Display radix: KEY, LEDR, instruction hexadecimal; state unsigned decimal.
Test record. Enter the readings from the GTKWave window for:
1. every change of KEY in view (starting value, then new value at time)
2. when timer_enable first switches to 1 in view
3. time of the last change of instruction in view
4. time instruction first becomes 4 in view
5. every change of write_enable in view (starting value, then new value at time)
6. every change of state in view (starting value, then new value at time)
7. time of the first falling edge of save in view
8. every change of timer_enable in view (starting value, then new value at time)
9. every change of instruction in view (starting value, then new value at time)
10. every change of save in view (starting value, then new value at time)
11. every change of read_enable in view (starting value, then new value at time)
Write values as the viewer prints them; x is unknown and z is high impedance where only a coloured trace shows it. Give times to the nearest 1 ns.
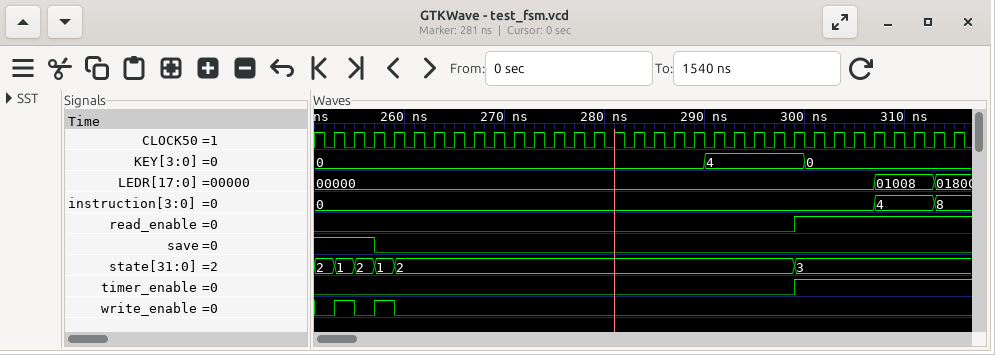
0, 4 at 290 ns, 0 at 300 ns
299 ns
313 ns
307 ns
0, 1 at 253 ns, 0 at 255 ns, 1 at 257 ns, 0 at 259 ns
2, 1 at 253 ns, 2 at 255 ns, 1 at 257 ns, 2 at 259 ns, 3 at 299 ns
257 ns
0, 1 at 299 ns
0, 4 at 307 ns, 8 at 313 ns
1, 0 at 257 ns
0, 1 at 299 ns
